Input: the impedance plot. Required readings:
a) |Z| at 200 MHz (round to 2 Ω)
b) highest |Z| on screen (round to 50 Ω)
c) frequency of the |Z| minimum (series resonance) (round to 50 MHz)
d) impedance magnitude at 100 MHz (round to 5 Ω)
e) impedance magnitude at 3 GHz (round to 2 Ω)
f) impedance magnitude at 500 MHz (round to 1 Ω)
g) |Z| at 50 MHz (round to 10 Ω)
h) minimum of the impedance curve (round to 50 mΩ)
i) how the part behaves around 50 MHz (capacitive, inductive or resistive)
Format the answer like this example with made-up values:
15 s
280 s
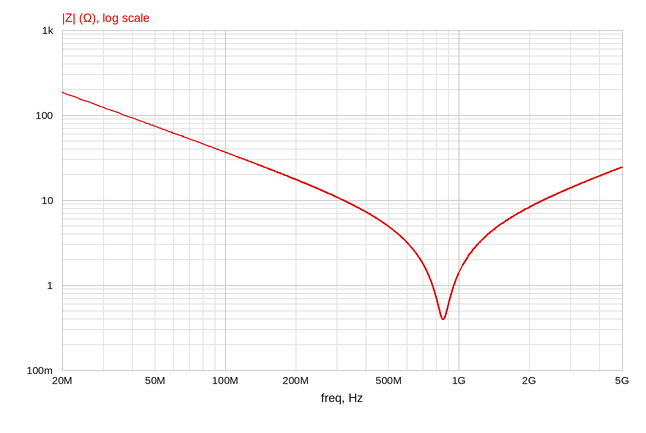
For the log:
18 Ω
200 Ω
850 MHz
35 Ω
14 Ω
5 Ω
70 Ω
400 mΩ
capacitive
